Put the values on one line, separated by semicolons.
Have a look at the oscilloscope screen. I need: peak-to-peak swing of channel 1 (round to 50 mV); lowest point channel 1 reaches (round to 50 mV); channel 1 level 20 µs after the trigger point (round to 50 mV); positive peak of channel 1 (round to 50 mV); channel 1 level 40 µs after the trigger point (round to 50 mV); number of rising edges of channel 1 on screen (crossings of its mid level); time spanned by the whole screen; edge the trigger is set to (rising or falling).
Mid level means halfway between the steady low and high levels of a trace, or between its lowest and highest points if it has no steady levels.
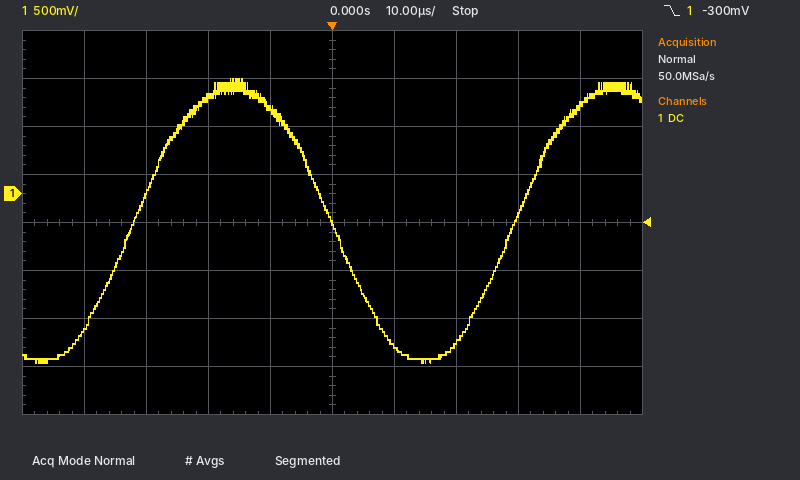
2.95 V; -1.75 V; -1.55 V; 1.20 V; 900 mV; 2; 100 µs; falling
